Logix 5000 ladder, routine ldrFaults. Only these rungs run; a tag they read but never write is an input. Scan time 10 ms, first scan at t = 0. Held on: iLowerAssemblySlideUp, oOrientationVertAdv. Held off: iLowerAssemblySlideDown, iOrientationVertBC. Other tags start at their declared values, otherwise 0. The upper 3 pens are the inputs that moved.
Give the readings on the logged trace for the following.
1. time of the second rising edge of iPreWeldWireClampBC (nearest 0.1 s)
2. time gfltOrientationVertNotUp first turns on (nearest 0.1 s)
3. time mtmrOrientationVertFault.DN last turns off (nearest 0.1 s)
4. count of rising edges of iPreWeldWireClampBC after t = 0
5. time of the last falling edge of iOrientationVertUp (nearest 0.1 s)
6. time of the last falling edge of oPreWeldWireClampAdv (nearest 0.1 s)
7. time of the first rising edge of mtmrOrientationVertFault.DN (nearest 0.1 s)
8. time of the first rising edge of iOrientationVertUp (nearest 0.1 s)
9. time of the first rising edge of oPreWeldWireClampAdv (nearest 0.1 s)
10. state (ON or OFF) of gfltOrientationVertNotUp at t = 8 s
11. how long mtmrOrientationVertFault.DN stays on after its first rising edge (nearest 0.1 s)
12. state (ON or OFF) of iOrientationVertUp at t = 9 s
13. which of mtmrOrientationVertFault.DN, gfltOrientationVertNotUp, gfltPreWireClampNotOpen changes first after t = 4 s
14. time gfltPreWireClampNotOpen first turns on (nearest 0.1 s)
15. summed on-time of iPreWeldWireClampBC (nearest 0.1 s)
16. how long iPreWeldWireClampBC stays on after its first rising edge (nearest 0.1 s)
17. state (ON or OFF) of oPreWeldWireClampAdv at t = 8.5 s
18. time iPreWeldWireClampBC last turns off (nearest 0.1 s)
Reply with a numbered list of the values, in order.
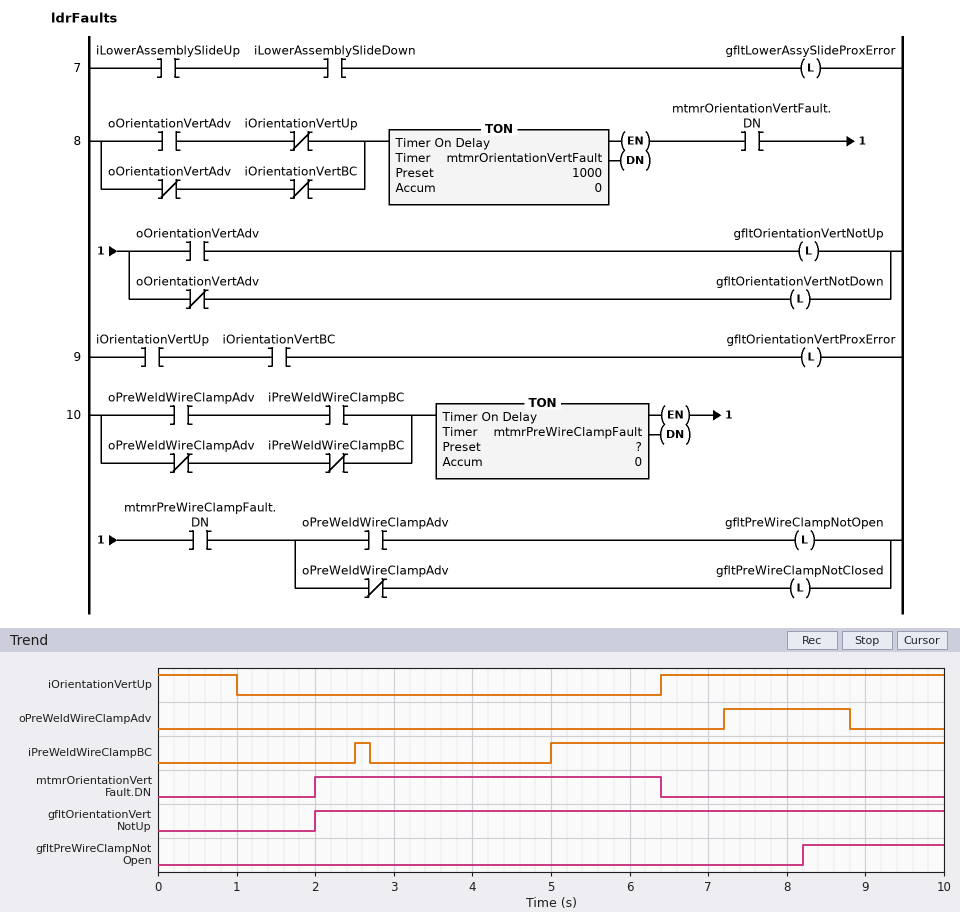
1. 5.0 s
2. 2.0 s
3. 6.4 s
4. 2
5. 1.0 s
6. 8.8 s
7. 2.0 s
8. 6.4 s
9. 7.2 s
10. ON
11. 4.4 s
12. ON
13. mtmrOrientationVertFault.DN
14. 8.2 s
15. 5.2 s
16. 0.2 s
17. ON
18. 2.7 s
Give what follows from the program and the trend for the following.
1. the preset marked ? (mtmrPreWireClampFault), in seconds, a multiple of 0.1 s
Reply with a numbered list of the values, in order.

1. 1.0 s
